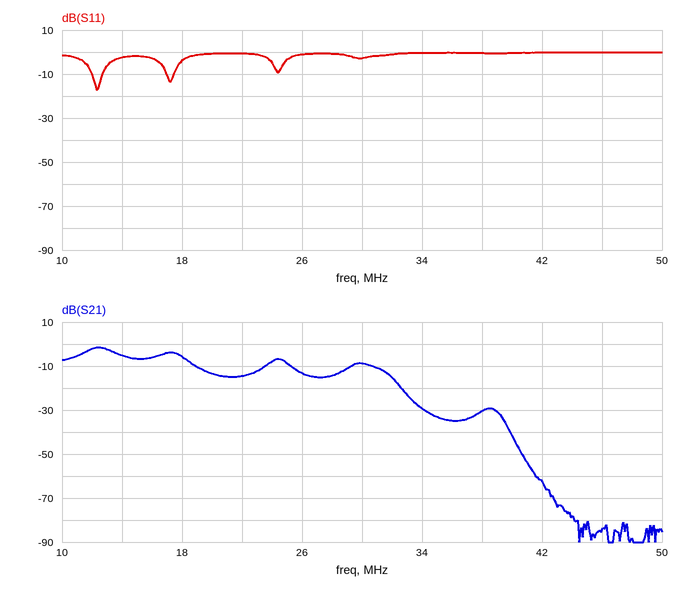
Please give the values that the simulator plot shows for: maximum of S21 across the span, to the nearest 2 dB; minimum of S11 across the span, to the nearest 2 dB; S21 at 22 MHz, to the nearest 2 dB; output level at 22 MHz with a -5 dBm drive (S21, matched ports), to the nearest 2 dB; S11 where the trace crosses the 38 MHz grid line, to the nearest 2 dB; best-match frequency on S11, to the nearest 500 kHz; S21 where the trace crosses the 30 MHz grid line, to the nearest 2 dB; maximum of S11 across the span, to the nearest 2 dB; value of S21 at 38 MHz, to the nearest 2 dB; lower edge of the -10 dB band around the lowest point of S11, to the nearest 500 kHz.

-2 dB
-18 dB
-14 dB
-20 dBm
0 dB
12.5 MHz
-8 dB
0 dB
-30 dB
12.0 MHz
